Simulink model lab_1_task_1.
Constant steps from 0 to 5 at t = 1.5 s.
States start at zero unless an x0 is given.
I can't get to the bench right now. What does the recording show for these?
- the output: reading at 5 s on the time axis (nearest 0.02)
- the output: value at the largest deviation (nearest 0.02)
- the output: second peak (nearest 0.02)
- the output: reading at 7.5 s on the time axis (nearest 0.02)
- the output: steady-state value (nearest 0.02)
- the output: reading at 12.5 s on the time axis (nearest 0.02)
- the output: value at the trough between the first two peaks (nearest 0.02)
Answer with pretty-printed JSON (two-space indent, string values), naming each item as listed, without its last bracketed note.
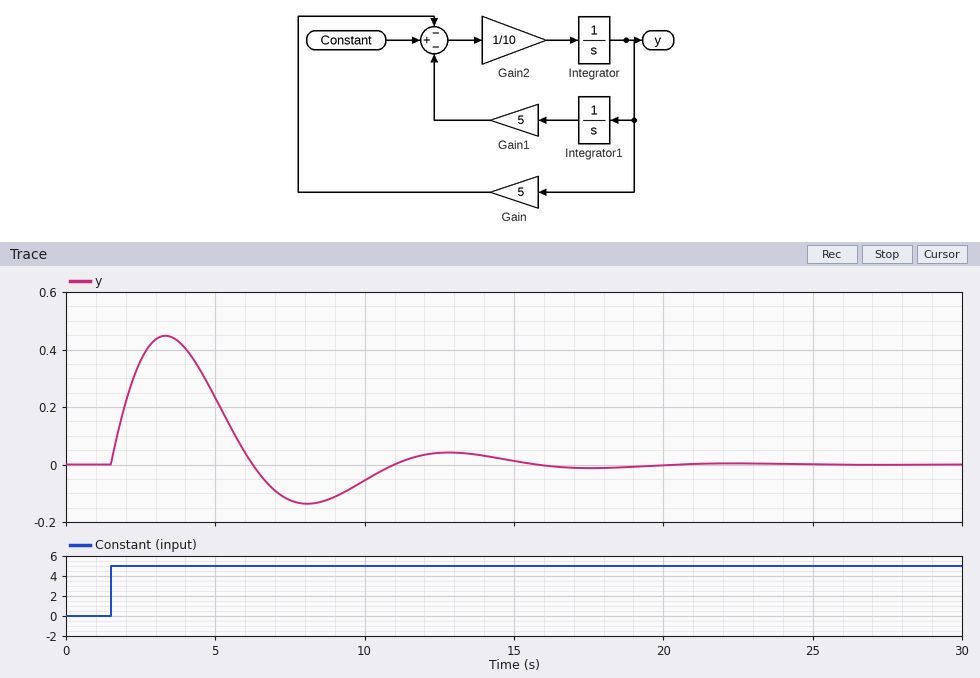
{
  "the output: reading at 5 s on the time axis": "0.24",
  "the output: value at the largest deviation": "0.44",
  "the output: second peak": "0.04",
  "the output: reading at 7.5 s on the time axis": "-0.12",
  "the output: steady-state value": "0.00",
  "the output: reading at 12.5 s on the time axis": "0.04",
  "the output: value at the trough between the first two peaks": "-0.14"
}
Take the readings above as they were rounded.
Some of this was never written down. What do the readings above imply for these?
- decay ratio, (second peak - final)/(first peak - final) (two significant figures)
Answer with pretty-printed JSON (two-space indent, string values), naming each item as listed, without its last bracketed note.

{
  "decay ratio, (second peak - final)/(first peak - final)": "0.091"
}
